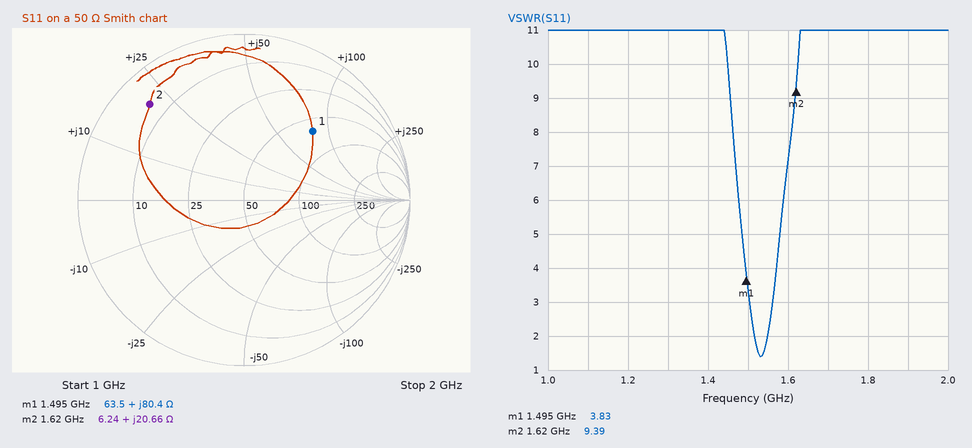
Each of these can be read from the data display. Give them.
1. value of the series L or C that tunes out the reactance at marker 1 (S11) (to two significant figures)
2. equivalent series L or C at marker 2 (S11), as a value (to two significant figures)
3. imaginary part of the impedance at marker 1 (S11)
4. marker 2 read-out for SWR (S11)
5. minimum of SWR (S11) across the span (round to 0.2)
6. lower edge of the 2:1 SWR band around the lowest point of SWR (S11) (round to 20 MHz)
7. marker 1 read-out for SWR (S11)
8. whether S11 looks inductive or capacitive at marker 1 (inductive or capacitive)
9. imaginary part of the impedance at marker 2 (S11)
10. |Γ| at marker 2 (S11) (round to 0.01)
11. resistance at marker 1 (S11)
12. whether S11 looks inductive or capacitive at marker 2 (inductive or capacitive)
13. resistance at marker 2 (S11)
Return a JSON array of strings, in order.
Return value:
["1.3 pF", "2.0 nH", "+80.4 Ω", "9.39", "1.4", "1.52 GHz", "3.83", "inductive", "+20.66 Ω", "0.81", "63.5 Ω", "inductive", "6.24 Ω"]
